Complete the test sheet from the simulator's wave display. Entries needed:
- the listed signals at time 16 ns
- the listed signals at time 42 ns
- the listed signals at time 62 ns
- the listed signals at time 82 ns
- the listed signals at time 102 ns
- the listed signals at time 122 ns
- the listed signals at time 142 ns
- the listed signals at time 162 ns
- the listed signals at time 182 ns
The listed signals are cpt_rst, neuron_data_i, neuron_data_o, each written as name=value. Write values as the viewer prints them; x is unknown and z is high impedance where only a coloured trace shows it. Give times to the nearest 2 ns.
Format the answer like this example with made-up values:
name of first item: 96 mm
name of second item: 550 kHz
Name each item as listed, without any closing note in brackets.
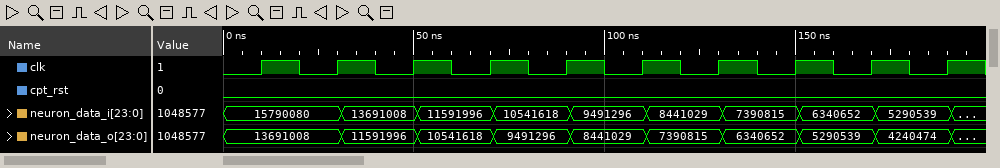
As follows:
the listed signals at time 16 ns: cpt_rst=0, neuron_data_i=15790080, neuron_data_o=13691008
the listed signals at time 42 ns: cpt_rst=0, neuron_data_i=13691008, neuron_data_o=11591996
the listed signals at time 62 ns: cpt_rst=0, neuron_data_i=11591996, neuron_data_o=10541618
the listed signals at time 82 ns: cpt_rst=0, neuron_data_i=10541618, neuron_data_o=9491296
the listed signals at time 102 ns: cpt_rst=0, neuron_data_i=9491296, neuron_data_o=8441029
the listed signals at time 122 ns: cpt_rst=0, neuron_data_i=8441029, neuron_data_o=7390815
the listed signals at time 142 ns: cpt_rst=0, neuron_data_i=7390815, neuron_data_o=6340652
the listed signals at time 162 ns: cpt_rst=0, neuron_data_i=6340652, neuron_data_o=5290539
the listed signals at time 182 ns: cpt_rst=0, neuron_data_i=5290539, neuron_data_o=4240474
